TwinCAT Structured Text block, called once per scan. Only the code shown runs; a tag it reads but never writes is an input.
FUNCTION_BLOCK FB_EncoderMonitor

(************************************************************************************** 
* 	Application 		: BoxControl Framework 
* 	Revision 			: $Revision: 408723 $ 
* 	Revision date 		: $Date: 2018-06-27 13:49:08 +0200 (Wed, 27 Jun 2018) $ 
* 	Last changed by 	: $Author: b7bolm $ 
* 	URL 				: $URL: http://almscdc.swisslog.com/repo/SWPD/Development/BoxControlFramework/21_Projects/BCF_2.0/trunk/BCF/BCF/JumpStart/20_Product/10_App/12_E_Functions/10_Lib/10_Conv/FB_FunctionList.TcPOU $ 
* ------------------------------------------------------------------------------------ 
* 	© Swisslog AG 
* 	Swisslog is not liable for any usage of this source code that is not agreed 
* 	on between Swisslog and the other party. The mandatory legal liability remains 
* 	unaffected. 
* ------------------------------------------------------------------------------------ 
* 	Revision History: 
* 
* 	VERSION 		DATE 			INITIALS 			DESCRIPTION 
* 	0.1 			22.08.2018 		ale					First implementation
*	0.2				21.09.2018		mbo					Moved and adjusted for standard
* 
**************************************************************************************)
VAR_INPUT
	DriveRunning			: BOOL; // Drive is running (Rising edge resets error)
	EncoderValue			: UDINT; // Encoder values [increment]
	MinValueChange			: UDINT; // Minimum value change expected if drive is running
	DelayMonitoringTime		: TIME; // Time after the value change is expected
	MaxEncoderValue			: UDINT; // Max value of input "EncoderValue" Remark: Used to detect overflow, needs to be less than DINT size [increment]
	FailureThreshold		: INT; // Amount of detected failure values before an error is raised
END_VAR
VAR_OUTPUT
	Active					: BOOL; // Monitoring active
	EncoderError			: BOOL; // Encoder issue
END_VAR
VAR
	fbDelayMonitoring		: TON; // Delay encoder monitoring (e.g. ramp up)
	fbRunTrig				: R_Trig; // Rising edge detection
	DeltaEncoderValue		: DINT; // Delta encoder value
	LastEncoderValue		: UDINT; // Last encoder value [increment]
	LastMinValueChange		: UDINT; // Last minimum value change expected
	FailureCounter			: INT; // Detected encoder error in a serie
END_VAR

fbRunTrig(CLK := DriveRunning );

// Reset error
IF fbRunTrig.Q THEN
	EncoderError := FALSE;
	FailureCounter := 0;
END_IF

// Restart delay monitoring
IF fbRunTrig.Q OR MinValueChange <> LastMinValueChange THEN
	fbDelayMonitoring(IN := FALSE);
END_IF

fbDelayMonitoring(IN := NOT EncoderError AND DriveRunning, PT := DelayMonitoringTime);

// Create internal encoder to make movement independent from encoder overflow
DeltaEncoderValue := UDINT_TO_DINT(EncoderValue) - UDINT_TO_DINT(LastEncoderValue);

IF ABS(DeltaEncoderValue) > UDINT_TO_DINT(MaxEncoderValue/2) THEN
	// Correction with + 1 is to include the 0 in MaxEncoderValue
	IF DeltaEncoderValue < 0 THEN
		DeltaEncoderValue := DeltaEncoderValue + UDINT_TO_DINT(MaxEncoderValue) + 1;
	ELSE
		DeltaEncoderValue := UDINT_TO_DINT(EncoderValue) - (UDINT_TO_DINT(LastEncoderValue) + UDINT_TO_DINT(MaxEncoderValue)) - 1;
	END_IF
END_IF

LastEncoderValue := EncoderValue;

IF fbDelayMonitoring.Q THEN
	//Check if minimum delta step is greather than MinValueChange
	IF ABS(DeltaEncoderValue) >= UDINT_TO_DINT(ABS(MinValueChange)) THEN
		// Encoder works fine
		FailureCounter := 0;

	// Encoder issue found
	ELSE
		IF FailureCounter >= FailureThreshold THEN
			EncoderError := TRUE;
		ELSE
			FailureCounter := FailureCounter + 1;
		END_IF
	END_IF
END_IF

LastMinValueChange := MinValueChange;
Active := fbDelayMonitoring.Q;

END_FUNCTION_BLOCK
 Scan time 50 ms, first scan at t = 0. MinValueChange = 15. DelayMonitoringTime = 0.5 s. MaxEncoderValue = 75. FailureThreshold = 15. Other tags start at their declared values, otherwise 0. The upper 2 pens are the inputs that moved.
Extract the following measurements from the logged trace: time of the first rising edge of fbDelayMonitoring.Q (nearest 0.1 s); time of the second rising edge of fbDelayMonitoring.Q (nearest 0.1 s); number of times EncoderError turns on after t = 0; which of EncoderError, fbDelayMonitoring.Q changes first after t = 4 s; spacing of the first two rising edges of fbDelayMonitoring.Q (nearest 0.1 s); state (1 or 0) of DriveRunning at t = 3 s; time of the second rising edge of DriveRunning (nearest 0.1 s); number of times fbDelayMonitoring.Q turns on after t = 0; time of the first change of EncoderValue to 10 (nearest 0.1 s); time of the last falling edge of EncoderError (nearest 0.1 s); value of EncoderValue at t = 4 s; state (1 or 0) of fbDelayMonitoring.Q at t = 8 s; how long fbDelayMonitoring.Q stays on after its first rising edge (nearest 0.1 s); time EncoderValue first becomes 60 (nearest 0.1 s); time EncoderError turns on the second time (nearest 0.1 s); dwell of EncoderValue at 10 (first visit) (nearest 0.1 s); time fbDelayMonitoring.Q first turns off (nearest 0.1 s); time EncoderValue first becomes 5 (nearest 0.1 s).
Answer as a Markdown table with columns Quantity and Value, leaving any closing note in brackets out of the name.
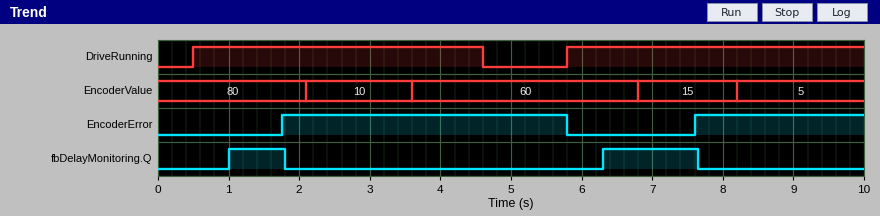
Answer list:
| Quantity | Value |
|---|---|
| time of the first rising edge of fbDelayMonitoring.Q | 1.0 s |
| time of the second rising edge of fbDelayMonitoring.Q | 6.3 s |
| number of times EncoderError turns on after t = 0 | 2 |
| which of EncoderError, fbDelayMonitoring.Q changes first after t = 4 s | EncoderError |
| spacing of the first two rising edges of fbDelayMonitoring.Q | 5.3 s |
| state (1 or 0) of DriveRunning at t = 3 s | 1 |
| time of the second rising edge of DriveRunning | 5.8 s |
| number of times fbDelayMonitoring.Q turns on after t = 0 | 2 |
| time of the first change of EncoderValue to 10 | 2.1 s |
| time of the last falling edge of EncoderError | 5.8 s |
| value of EncoderValue at t = 4 s | 60 |
| state (1 or 0) of fbDelayMonitoring.Q at t = 8 s | 0 |
| how long fbDelayMonitoring.Q stays on after its first rising edge | 0.8 s |
| time EncoderValue first becomes 60 | 3.6 s |
| time EncoderError turns on the second time | 7.6 s |
| dwell of EncoderValue at 10 (first visit) | 1.5 s |
| time fbDelayMonitoring.Q first turns off | 1.8 s |
| time EncoderValue first becomes 5 | 8.2 s |
